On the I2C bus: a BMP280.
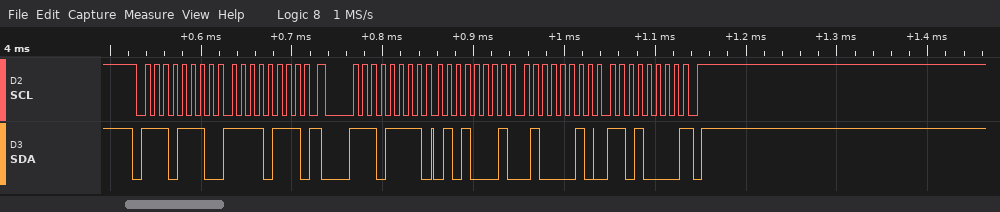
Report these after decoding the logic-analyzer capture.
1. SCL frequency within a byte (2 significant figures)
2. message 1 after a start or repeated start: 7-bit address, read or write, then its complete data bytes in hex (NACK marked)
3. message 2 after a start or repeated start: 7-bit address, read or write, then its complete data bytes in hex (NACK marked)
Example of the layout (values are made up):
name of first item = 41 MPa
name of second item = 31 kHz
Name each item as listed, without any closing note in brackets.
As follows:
SCL frequency within a byte = 100 kHz
message 1 after a start or repeated start: 7-bit address, read or write, then its complete data bytes in hex = 0x77 write: F7
message 2 after a start or repeated start: 7-bit address, read or write, then its complete data bytes in hex = 0x77 read: 51 42 D0 NACK
